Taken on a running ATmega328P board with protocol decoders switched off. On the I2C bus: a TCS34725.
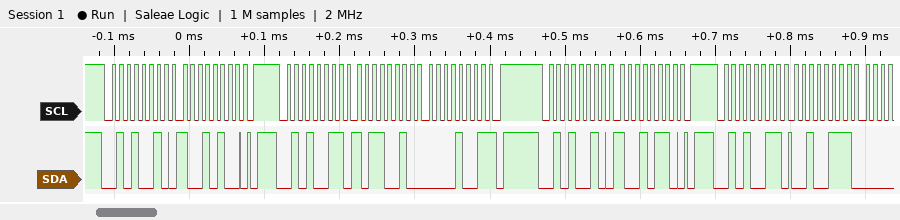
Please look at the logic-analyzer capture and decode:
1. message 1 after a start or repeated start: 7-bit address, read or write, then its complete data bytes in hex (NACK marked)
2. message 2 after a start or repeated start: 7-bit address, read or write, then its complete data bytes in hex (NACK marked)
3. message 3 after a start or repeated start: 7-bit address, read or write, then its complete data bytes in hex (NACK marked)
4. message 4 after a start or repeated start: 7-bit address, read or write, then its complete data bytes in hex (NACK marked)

0x29 write: 94
0x29 read: B2 09 NACK
0x29 write: 96
0x29 read: 27
